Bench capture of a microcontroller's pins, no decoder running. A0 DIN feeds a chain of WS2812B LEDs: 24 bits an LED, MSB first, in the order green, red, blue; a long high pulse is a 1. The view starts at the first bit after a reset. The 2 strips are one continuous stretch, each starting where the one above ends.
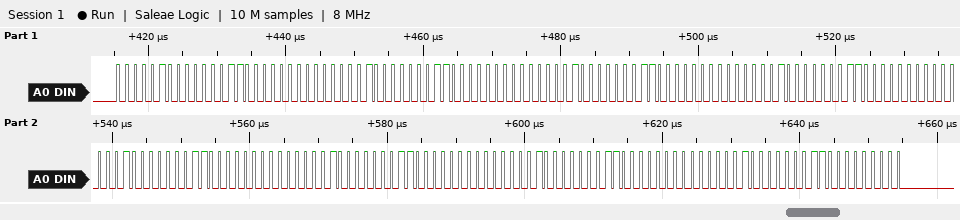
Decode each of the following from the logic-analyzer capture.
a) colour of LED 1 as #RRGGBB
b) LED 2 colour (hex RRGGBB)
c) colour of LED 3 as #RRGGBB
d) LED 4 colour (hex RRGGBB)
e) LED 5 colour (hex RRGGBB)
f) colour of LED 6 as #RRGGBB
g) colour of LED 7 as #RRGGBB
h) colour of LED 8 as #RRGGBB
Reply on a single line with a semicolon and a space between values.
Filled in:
#060400; #060400; #060400; #060400; #060400; #060400; #060400; #060400
